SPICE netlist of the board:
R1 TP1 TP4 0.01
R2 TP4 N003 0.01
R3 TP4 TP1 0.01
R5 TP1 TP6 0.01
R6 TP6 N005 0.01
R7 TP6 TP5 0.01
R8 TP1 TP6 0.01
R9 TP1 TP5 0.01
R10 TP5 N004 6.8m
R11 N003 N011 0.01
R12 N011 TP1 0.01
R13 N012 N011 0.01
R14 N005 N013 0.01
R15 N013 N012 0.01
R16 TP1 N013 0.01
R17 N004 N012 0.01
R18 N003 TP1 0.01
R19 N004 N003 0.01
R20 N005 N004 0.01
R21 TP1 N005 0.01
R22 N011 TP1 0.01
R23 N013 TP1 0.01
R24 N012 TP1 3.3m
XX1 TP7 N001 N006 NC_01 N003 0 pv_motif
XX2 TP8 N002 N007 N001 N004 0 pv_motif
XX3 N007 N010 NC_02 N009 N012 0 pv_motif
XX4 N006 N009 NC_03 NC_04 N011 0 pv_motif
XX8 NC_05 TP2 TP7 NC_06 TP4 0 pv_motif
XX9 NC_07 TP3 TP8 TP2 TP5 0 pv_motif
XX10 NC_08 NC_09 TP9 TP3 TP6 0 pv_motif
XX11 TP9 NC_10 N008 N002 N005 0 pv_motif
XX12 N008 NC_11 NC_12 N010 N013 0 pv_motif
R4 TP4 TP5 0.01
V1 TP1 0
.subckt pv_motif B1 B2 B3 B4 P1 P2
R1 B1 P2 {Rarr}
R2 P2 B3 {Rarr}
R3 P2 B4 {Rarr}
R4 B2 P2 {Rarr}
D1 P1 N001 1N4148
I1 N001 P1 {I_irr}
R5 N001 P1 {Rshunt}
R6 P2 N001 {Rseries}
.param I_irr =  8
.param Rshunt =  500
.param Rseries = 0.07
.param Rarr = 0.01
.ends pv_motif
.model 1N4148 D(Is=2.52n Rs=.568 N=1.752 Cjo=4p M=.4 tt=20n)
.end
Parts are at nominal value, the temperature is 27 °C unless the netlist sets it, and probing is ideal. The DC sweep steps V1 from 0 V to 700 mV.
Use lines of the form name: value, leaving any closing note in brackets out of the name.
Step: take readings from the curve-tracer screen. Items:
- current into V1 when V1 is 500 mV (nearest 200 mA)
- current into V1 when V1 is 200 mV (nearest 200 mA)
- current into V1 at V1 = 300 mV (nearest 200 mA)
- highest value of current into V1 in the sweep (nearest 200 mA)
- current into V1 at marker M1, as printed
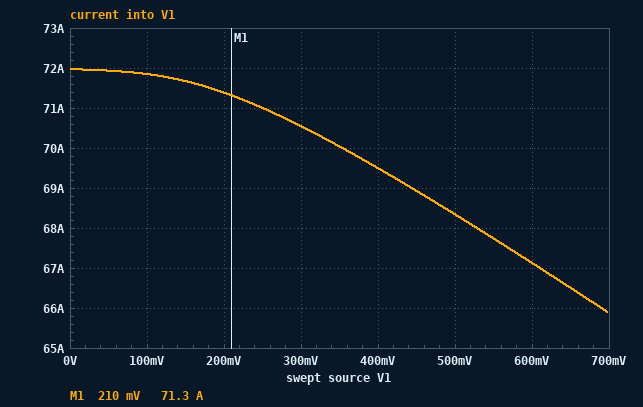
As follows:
current into V1 when V1 is 500 mV: 68.4 A
current into V1 when V1 is 200 mV: 71.4 A
current into V1 at V1 = 300 mV: 70.6 A
highest value of current into V1 in the sweep: 72.0 A
current into V1 at marker M1, as printed: 71.3 A
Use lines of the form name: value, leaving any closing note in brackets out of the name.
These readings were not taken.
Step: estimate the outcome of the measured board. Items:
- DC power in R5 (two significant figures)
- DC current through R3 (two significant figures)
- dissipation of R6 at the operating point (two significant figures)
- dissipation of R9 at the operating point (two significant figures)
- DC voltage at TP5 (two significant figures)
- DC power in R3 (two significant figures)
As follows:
DC power in R5: 280 mW
DC current through R3: 5.3 A
dissipation of R6 at the operating point: 13 mW
dissipation of R9 at the operating point: 450 mW
DC voltage at TP5: 67 mV
DC power in R3: 280 mW
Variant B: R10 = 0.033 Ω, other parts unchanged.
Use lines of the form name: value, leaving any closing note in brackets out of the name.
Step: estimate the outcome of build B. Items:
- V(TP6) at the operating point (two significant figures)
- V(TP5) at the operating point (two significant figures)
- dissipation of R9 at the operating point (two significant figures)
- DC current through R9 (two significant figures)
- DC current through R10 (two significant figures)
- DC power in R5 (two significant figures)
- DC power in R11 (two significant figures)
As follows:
V(TP6) at the operating point: 52 mV
V(TP5) at the operating point: 63 mV
dissipation of R9 at the operating point: 400 mW
DC current through R9: 6.3 A
DC current through R10: 580 mA
DC power in R5: 270 mW
DC power in R11: 34 mW
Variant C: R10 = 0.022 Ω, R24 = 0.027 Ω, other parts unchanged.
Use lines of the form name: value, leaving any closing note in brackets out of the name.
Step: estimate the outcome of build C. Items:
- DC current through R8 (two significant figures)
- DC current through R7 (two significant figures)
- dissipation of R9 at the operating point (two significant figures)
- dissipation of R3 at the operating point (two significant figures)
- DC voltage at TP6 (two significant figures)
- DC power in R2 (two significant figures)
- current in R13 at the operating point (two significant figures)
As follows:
DC current through R8: 5.6 A
DC current through R7: 1.3 A
dissipation of R9 at the operating point: 470 mW
dissipation of R3 at the operating point: 310 mW
DC voltage at TP6: 56 mV
DC power in R2: 35 mW
current in R13 at the operating point: 2.9 A
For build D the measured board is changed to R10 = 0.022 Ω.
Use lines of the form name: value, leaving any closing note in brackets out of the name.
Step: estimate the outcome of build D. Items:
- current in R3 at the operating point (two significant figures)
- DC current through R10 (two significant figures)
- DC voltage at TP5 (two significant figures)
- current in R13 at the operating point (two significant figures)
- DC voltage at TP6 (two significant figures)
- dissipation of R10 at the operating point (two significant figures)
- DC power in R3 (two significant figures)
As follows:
current in R3 at the operating point: 5.2 A
DC current through R10: 790 mA
DC voltage at TP5: 64 mV
current in R13 at the operating point: 450 mA
DC voltage at TP6: 52 mV
dissipation of R10 at the operating point: 14 mW
DC power in R3: 270 mW
